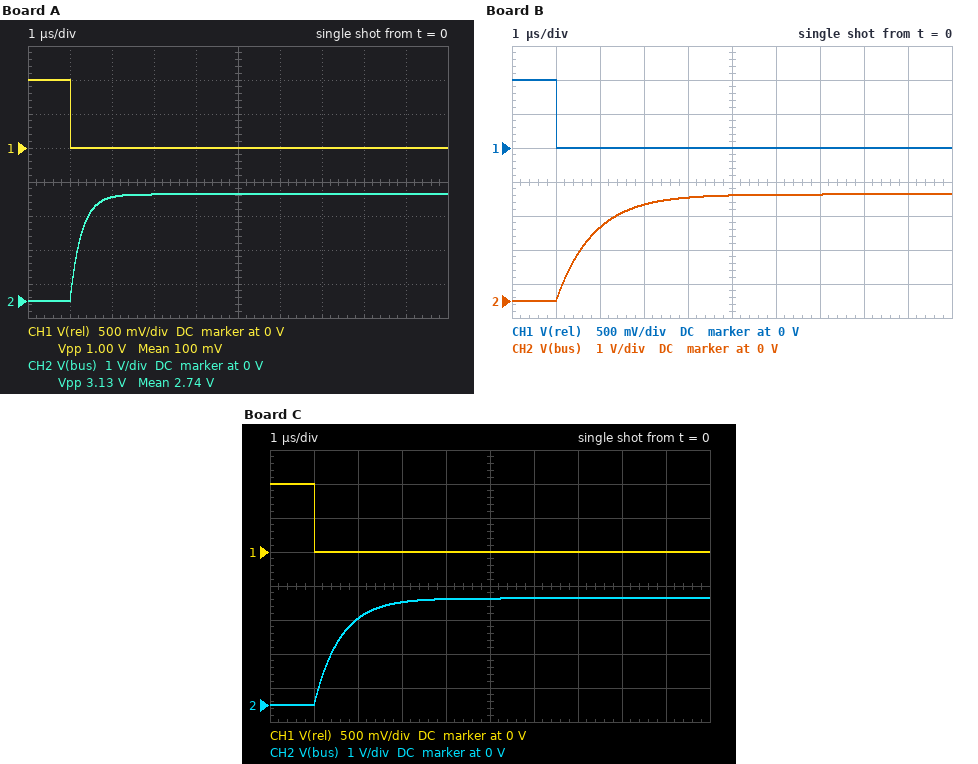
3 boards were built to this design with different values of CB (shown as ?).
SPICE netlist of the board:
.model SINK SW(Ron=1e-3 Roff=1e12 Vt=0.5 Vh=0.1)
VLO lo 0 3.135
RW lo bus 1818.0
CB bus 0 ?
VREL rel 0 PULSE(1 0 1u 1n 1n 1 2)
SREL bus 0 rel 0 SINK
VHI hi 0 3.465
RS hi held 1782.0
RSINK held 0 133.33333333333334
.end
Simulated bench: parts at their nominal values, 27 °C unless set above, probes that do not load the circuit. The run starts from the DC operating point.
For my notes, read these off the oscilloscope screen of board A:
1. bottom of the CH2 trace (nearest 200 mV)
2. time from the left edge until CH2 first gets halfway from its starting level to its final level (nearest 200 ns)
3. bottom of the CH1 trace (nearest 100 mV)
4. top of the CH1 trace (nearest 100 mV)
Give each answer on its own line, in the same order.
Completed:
0 V
1.2 µs
0 V
1.0 V
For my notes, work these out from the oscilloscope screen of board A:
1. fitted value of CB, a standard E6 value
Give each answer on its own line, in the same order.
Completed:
150 pF
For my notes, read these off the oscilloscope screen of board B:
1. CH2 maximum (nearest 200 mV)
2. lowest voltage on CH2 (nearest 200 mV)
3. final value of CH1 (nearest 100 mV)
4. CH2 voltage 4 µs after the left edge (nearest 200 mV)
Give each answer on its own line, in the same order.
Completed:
3.2 V
0 V
0 V
3.0 V
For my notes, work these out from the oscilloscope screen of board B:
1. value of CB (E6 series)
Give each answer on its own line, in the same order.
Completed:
470 pF
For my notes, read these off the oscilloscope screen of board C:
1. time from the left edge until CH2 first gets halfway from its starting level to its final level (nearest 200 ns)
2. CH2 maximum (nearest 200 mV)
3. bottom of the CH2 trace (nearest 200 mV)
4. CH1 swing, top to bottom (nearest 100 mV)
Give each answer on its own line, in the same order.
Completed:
1.4 µs
3.2 V
0 V
1.0 V
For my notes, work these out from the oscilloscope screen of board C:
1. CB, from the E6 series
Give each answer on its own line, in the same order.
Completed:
330 pF
